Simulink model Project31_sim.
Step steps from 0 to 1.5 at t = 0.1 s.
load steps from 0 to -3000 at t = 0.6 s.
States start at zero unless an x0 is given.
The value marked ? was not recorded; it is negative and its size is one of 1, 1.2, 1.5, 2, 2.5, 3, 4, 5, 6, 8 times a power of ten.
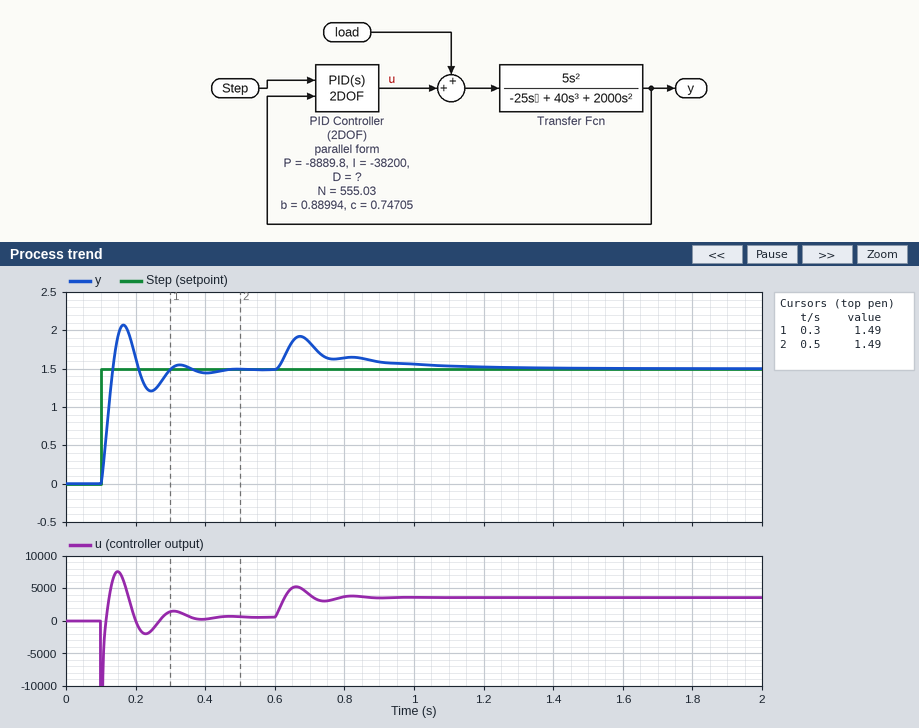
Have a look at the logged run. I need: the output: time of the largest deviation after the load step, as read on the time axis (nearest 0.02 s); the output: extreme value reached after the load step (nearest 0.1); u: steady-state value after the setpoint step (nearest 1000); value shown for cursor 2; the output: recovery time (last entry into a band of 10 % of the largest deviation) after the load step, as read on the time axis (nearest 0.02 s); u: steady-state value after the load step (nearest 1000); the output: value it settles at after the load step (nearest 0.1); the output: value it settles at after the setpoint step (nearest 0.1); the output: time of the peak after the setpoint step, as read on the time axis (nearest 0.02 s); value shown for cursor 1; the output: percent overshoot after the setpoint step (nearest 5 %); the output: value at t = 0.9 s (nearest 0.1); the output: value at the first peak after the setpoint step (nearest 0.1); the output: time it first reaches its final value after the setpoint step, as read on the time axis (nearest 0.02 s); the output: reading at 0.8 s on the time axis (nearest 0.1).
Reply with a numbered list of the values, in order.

1. 0.68 s
2. 1.9
3. 1000
4. 1.49
5. 1.06 s
6. 4000
7. 1.5
8. 1.5
9. 0.16 s
10. 1.49
11. 40 %
12. 1.6
13. 2.1
14. 0.14 s
15. 1.6
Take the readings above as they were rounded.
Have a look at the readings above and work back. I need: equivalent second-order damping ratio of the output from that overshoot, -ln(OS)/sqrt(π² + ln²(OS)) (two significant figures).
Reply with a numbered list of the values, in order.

1. 0.28
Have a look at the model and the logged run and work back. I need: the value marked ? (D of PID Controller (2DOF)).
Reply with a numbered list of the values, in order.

1. -150
